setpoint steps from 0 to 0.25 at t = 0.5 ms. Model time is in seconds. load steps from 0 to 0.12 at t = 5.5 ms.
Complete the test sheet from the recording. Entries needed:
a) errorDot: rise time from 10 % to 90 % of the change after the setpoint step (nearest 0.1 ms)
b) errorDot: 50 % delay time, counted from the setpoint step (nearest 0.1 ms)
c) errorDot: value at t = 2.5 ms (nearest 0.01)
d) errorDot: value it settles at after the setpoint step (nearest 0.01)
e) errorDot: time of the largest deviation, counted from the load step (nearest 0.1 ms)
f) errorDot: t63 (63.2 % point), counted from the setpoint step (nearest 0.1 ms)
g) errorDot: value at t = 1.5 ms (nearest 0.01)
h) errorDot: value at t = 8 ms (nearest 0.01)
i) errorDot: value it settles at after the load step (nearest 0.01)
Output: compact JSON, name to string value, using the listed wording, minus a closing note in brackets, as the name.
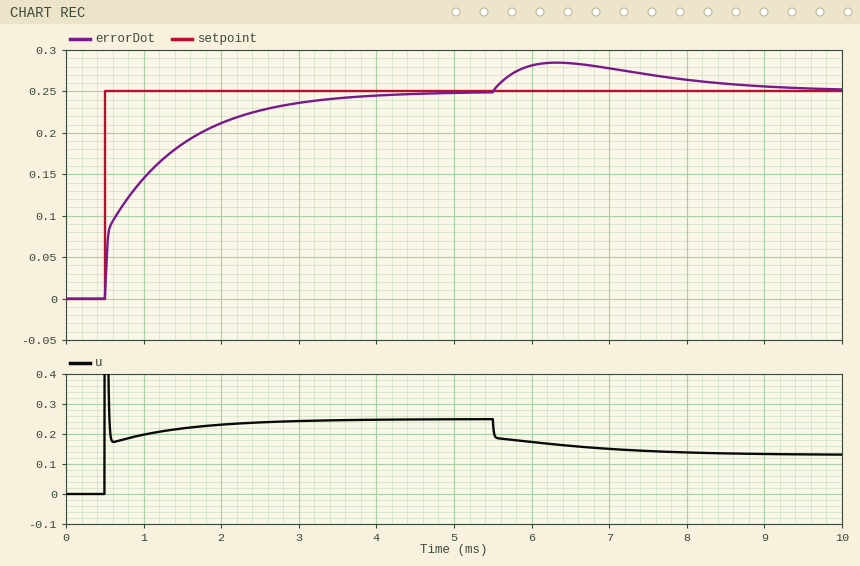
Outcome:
{"errorDot: rise time from 10 % to 90 % of the change after the setpoint step": "1.9 ms", "errorDot: 50 % delay time, counted from the setpoint step": "0.3 ms", "errorDot: value at t = 2.5 ms": "0.23", "errorDot: value it settles at after the setpoint step": "0.25", "errorDot: time of the largest deviation, counted from the load step": "0.8 ms", "errorDot: t63 (63.2 % point), counted from the setpoint step": "0.6 ms", "errorDot: value at t = 1.5 ms": "0.19", "errorDot: value at t = 8 ms": "0.26", "errorDot: value it settles at after the load step": "0.25"}
